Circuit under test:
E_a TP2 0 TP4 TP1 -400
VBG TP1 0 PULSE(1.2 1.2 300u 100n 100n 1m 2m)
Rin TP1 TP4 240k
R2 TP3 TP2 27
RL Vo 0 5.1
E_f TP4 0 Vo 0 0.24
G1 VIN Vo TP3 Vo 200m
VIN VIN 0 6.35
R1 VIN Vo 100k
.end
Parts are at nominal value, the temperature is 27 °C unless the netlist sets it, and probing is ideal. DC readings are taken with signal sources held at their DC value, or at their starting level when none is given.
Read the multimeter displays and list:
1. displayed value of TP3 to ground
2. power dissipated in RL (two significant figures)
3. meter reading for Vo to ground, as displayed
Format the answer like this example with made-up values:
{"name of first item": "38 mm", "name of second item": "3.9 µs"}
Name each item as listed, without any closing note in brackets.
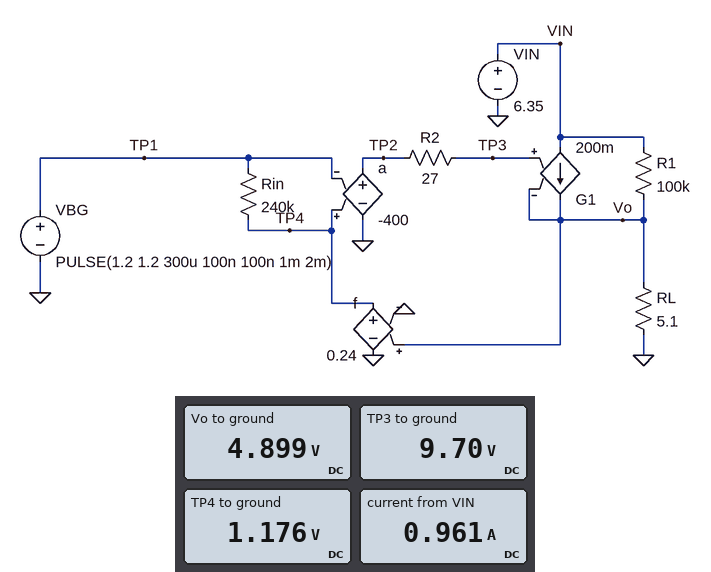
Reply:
{"displayed value of TP3 to ground": "9.70 V", "power dissipated in RL": "4.7 W", "meter reading for Vo to ground, as displayed": "4.899 V"}
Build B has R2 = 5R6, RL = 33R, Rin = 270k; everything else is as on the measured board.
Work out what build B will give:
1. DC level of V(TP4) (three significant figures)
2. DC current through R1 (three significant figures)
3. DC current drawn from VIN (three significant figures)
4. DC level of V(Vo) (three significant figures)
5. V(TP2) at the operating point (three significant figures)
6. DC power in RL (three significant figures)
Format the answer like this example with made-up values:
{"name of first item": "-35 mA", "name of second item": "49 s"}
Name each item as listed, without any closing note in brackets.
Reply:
{"DC level of V(TP4)": "1.19 V", "DC current through R1": "14.1 µA", "DC current drawn from VIN": "150 mA", "DC level of V(Vo)": "4.94 V", "V(TP2) at the operating point": "5.69 V", "DC power in RL": "740 mW"}
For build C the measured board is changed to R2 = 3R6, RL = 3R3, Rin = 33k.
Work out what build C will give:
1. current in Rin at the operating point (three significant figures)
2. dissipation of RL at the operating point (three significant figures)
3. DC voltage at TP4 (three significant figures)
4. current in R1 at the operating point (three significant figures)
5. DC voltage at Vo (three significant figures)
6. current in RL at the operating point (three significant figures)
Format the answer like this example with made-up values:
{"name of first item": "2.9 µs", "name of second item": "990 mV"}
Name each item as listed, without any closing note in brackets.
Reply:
{"current in Rin at the operating point": "928 nA", "dissipation of RL at the operating point": "7.19 W", "DC voltage at TP4": "1.17 V", "current in R1 at the operating point": "14.8 µA", "DC voltage at Vo": "4.87 V", "current in RL at the operating point": "1.48 A"}
